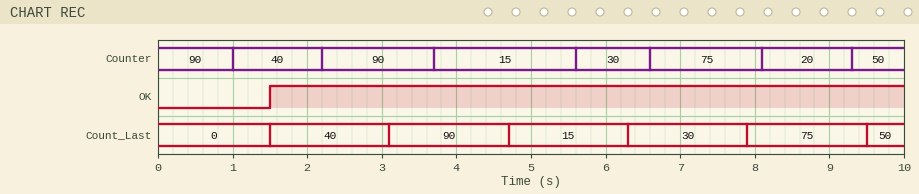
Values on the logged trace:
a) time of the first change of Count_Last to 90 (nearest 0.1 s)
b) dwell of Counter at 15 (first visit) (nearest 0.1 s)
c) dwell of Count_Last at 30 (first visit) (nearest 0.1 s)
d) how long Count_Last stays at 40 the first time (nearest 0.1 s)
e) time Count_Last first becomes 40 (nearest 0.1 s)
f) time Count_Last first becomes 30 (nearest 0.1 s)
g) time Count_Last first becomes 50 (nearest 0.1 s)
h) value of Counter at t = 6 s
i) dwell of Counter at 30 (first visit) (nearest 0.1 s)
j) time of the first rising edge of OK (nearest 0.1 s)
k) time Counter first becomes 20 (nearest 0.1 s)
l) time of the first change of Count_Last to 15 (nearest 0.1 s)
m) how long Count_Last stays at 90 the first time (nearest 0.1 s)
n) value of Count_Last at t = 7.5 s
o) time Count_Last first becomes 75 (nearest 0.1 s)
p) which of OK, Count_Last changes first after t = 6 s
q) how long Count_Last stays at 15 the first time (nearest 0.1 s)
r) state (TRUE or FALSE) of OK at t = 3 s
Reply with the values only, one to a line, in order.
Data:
3.1 s
1.9 s
1.6 s
1.6 s
1.5 s
6.3 s
9.5 s
30
1.0 s
1.5 s
8.1 s
4.7 s
1.6 s
30
7.9 s
Count_Last
1.6 s
TRUE
